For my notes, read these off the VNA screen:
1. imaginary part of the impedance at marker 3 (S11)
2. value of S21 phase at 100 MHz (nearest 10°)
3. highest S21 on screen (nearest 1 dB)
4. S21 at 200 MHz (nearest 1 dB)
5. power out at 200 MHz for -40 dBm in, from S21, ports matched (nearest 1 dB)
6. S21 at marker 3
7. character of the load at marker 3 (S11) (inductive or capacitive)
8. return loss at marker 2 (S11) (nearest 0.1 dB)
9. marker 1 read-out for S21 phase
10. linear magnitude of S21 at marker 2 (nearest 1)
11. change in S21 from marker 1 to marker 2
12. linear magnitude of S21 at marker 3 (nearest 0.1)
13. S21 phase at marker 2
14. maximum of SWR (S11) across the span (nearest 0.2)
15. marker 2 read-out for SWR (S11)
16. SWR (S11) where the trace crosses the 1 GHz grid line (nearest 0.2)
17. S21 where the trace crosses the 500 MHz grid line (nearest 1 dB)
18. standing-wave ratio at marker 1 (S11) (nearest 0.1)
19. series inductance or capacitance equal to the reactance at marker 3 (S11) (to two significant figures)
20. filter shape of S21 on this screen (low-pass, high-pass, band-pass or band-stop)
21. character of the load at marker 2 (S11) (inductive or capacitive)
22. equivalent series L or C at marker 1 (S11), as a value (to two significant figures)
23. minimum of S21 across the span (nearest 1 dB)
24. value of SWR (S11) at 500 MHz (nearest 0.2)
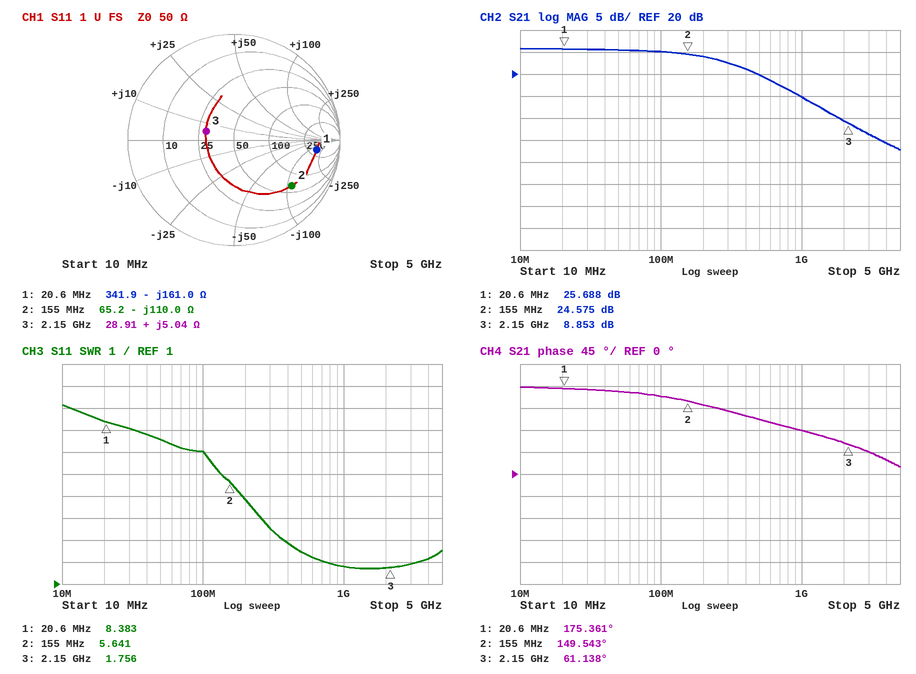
+5.04 Ω
160°
26 dB
24 dB
-16 dBm
8.853 dB
inductive
3.1 dB
175.361°
17
-1.113 dB
2.8
149.543°
9.2
5.641
1.8
20 dB
8.4
370 pH
low-pass
capacitive
48 pF
3 dB
2.4
